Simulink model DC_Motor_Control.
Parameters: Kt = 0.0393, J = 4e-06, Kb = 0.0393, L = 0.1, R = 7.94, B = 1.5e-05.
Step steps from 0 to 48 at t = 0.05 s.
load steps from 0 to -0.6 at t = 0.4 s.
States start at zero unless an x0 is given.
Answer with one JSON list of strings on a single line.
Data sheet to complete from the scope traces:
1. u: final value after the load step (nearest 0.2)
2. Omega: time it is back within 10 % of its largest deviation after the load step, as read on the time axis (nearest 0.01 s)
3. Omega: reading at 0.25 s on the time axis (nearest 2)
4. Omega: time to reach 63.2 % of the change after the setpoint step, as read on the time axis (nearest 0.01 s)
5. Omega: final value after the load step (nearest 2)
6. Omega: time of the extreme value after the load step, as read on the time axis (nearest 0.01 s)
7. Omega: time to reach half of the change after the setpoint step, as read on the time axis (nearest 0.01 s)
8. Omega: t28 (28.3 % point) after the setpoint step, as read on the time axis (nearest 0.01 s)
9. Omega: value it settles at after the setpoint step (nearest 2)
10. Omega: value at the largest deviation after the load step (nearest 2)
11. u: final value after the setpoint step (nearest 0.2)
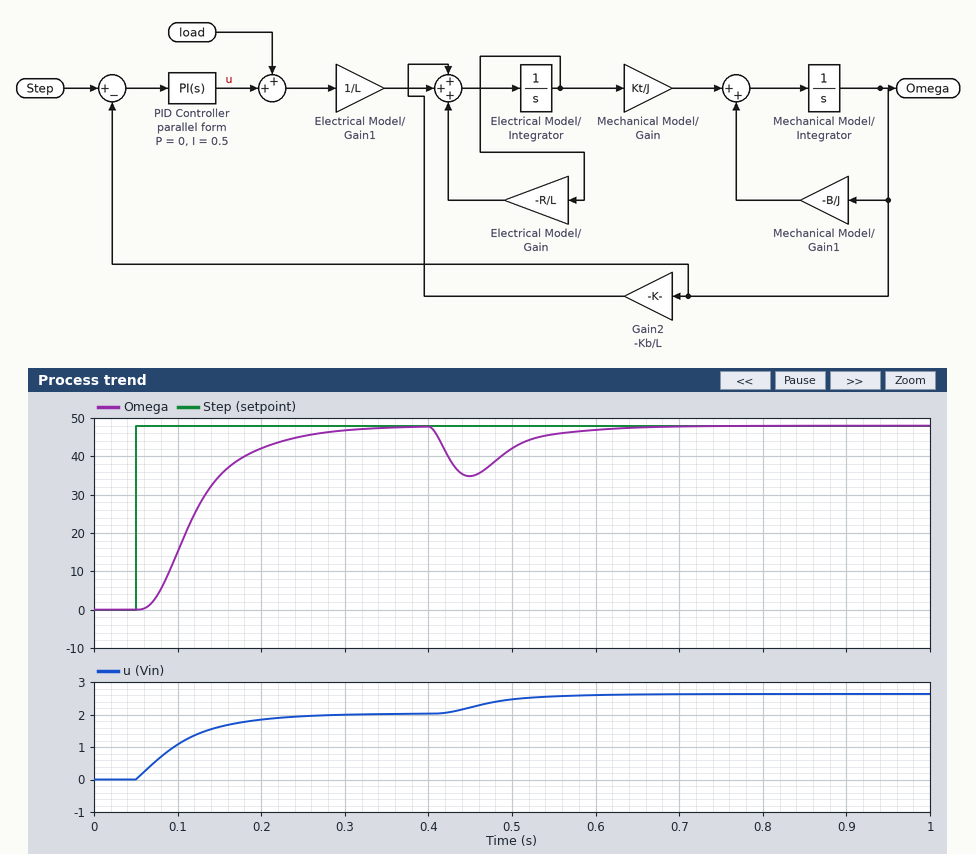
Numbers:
["2.6", "0.59 s", "46", "0.13 s", "48", "0.45 s", "0.12 s", "0.10 s", "48", "34", "2.0"]
